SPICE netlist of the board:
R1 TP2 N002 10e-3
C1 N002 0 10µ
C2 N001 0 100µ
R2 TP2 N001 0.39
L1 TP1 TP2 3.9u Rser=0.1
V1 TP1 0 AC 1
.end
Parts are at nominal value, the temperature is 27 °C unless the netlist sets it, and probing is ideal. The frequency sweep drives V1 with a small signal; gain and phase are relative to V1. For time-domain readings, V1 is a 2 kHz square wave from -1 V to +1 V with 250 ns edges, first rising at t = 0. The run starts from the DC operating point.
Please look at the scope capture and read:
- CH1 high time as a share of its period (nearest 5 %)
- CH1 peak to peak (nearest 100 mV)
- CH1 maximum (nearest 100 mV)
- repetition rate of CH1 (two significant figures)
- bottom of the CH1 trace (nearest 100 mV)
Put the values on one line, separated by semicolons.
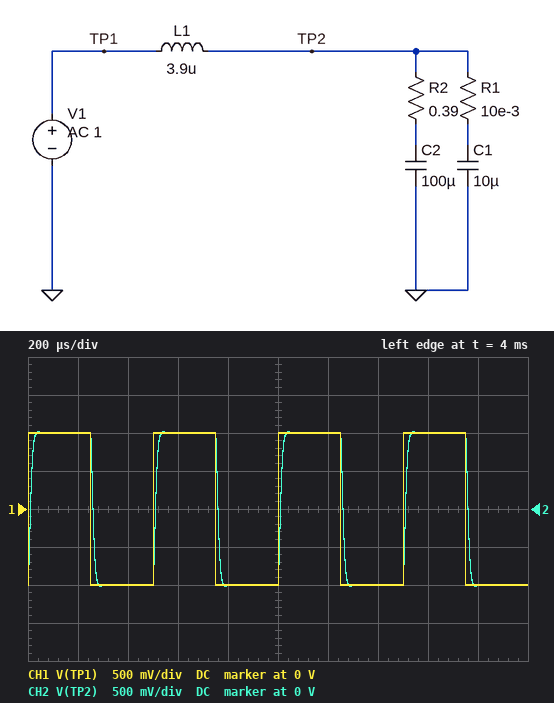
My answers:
50 %; 2.0 V; 1.0 V; 2.0 kHz; -1.0 V
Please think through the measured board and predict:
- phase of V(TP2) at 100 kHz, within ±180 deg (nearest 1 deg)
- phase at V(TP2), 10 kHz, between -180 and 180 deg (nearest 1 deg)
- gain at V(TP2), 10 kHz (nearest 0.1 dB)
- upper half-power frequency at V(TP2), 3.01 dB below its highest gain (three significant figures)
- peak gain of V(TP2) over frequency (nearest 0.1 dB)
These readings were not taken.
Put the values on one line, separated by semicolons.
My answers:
-151 deg; -39 deg; -0.8 dB; 19.4 kHz; 0 dB
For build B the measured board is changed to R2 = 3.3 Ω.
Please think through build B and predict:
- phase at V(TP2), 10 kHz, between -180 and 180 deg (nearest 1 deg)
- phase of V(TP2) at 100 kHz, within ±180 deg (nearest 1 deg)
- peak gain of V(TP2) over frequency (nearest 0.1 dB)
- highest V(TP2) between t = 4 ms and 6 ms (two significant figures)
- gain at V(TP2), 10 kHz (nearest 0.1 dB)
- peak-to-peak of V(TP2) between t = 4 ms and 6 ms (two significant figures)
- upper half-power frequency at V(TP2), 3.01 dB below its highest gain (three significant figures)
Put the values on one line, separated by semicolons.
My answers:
-9 deg; -171 deg; 8.8 dB; 2.1 V; 1.1 dB; 4.1 V; 29.3 kHz
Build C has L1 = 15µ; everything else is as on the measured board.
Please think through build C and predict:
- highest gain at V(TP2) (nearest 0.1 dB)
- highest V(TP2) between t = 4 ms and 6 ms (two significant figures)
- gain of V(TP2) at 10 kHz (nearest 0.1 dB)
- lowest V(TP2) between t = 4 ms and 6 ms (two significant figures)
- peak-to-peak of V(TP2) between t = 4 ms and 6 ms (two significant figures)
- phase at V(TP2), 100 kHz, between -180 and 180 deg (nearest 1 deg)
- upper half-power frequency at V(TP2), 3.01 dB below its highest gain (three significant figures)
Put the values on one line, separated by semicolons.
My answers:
2.0 dB; 1.4 V; -7.0 dB; -1.4 V; 2.8 V; -154 deg; 5.73 kHz
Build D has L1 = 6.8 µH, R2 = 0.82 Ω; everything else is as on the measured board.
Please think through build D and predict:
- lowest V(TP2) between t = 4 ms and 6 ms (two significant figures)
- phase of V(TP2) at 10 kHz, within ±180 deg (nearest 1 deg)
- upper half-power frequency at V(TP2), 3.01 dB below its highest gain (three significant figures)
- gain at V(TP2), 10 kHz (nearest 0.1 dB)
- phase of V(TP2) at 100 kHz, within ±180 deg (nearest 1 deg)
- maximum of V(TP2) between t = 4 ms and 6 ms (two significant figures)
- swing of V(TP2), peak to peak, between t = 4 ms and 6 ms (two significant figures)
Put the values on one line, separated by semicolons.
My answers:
-1.2 V; -38 deg; 22.1 kHz; 0.4 dB; -164 deg; 1.2 V; 2.4 V
